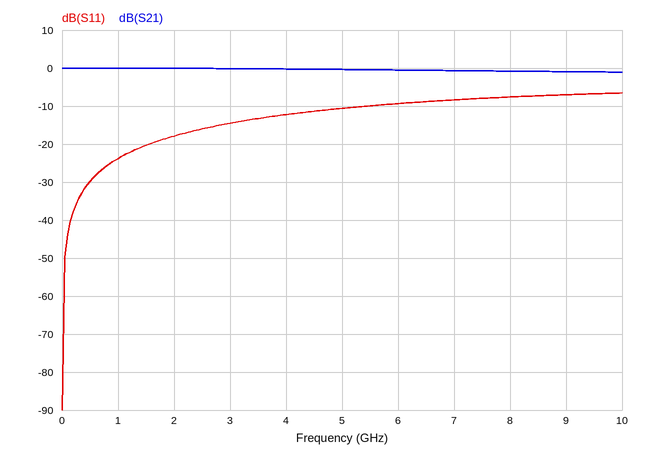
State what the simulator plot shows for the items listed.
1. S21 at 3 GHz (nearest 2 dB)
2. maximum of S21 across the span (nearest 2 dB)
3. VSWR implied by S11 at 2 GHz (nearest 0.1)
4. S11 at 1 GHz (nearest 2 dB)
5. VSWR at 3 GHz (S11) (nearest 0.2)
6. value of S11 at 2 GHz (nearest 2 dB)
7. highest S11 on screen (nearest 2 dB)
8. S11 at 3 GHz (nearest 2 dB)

0 dB
0 dB
1.3
-24 dB
1.4
-18 dB
-6 dB
-14 dB
